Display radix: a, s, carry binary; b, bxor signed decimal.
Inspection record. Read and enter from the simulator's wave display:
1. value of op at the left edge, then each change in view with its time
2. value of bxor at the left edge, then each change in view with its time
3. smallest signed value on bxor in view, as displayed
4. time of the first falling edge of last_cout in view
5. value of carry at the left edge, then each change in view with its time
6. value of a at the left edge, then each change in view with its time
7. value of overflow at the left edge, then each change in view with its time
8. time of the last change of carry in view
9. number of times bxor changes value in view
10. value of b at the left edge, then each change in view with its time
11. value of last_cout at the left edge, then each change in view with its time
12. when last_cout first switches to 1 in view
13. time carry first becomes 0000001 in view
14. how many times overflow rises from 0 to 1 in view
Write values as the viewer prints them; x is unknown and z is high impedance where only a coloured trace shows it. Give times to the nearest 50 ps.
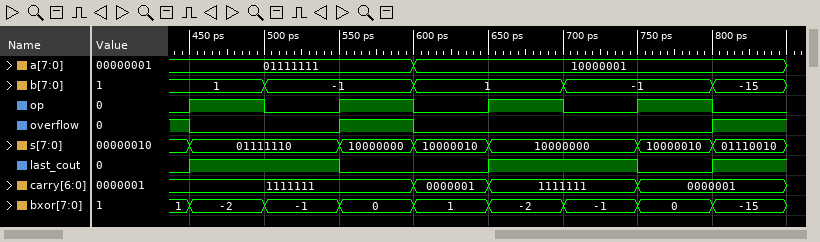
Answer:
0, 1 at 450 ps, 0 at 500 ps, 1 at 550 ps, 0 at 600 ps, 1 at 650 ps, 0 at 700 ps, 1 at 750 ps, 0 at 800 ps
1, -2 at 450 ps, -1 at 500 ps, 0 at 550 ps, 1 at 600 ps, -2 at 650 ps, -1 at 700 ps, 0 at 750 ps, -15 at 800 ps
-15
550 ps
1111111, 0000001 at 600 ps, 1111111 at 650 ps, 0000001 at 750 ps
01111111, 10000001 at 600 ps
1, 0 at 450 ps, 1 at 550 ps, 0 at 600 ps, 1 at 800 ps
750 ps
8
1, -1 at 500 ps, 1 at 600 ps, -1 at 700 ps, -15 at 800 ps
0, 1 at 450 ps, 0 at 550 ps, 1 at 650 ps, 0 at 750 ps, 1 at 800 ps
450 ps
600 ps
2
